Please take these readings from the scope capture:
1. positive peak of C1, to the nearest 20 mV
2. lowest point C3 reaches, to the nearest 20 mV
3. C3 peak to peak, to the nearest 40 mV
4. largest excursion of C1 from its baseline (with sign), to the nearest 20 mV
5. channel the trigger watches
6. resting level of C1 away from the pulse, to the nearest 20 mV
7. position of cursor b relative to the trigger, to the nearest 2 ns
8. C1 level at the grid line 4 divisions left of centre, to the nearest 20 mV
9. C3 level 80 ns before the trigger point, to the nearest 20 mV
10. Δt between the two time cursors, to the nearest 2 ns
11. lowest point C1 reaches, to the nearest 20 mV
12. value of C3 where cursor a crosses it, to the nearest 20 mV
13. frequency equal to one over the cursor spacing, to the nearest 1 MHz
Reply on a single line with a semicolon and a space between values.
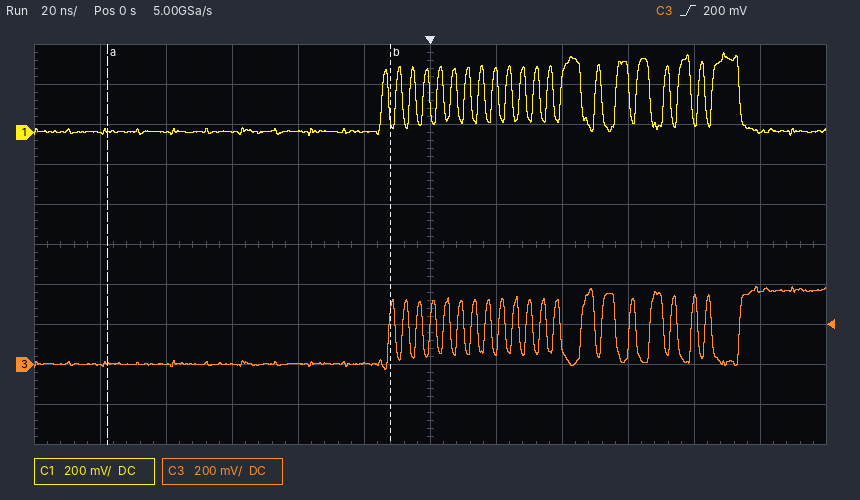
400 mV; -20 mV; 400 mV; +400 mV; C3; 0 mV; -12 ns; 0 mV; 0 mV; 86 ns; -20 mV; 0 mV; 12 MHz
